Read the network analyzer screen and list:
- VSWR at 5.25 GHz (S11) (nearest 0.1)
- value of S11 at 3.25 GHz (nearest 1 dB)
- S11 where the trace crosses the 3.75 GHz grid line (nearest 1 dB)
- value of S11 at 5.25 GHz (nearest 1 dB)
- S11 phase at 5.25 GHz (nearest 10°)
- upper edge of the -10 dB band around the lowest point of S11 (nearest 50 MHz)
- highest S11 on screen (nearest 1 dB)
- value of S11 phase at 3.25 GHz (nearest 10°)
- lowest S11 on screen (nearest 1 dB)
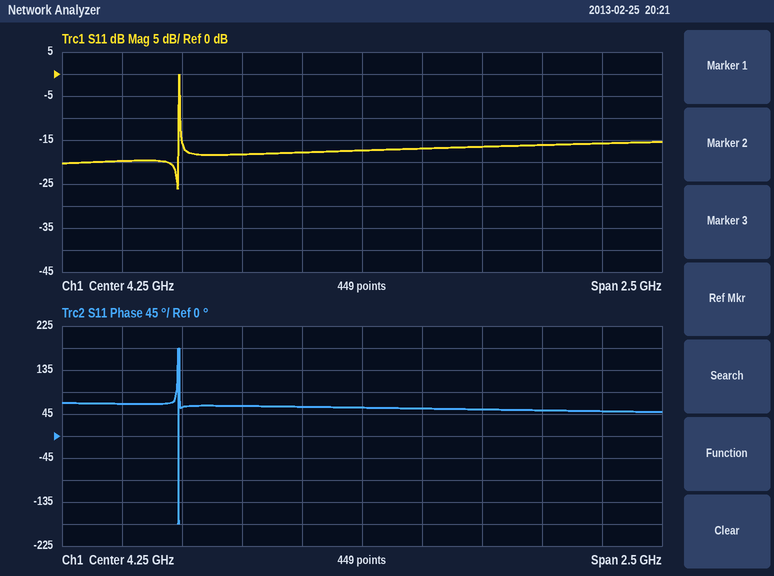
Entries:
1.4
-20 dB
-18 dB
-16 dB
50°
3.50 GHz
0 dB
70°
-26 dB
